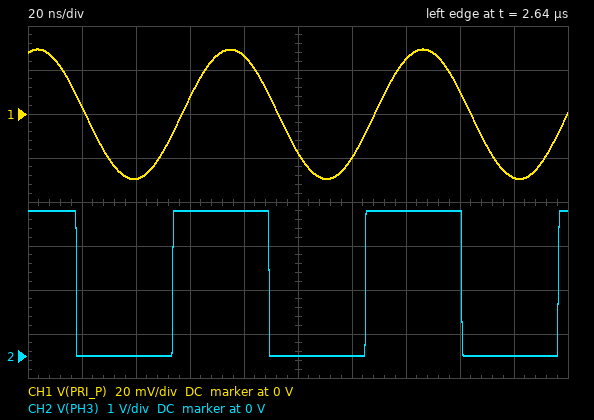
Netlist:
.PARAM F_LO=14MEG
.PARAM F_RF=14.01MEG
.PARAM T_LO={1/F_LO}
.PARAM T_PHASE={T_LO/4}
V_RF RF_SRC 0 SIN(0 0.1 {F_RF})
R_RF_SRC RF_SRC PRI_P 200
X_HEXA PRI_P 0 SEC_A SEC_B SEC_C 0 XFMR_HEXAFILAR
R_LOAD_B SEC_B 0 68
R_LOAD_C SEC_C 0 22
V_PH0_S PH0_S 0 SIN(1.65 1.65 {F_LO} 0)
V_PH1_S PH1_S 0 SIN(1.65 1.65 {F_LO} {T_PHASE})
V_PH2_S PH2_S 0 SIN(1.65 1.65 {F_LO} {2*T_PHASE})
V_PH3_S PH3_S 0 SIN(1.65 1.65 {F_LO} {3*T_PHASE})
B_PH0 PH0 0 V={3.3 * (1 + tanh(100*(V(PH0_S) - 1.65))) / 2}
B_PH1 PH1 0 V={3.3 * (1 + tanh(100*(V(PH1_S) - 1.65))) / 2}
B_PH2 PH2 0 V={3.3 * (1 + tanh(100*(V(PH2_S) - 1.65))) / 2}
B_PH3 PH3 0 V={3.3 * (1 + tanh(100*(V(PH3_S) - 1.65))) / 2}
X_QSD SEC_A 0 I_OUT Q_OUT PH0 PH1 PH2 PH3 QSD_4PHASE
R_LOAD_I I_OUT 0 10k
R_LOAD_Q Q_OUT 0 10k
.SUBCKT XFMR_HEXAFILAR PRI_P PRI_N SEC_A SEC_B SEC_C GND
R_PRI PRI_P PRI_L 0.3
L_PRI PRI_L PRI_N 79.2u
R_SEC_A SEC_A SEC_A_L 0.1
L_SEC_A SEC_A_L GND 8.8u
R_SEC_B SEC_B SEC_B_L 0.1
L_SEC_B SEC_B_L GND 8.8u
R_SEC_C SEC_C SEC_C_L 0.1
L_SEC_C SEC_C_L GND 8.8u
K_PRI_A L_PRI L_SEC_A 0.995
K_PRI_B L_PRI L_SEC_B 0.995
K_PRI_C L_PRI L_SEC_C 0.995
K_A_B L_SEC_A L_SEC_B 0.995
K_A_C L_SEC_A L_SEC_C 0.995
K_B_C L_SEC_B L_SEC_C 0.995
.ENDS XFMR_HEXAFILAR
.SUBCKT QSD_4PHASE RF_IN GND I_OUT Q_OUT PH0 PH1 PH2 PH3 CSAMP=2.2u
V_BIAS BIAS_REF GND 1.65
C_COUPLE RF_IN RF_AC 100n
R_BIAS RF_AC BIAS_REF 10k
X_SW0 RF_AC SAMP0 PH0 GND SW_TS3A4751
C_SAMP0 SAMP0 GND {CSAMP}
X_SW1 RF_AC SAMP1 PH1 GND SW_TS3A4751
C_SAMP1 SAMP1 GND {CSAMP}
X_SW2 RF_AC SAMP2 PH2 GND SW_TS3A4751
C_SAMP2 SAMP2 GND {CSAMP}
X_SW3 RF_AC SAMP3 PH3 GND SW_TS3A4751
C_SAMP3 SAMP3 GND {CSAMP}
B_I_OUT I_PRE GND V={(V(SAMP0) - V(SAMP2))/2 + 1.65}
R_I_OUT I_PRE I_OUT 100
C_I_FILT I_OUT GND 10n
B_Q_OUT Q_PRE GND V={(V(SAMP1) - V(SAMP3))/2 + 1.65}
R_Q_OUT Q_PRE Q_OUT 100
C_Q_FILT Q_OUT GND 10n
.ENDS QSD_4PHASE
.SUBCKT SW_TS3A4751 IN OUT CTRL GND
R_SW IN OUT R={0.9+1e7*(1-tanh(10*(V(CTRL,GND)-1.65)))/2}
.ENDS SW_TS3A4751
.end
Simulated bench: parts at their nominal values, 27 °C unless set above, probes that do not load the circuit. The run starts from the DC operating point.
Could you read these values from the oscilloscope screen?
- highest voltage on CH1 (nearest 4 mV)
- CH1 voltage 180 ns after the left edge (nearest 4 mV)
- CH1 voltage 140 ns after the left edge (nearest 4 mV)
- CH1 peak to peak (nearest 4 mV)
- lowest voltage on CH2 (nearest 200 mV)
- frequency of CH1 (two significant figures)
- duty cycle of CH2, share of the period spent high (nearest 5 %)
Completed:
28 mV
-28 mV
24 mV
60 mV
0 V
14 MHz
50 %
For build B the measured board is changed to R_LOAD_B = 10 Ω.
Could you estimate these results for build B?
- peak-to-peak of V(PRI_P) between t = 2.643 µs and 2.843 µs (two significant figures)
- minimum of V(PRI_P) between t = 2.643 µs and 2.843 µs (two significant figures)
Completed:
53 mV
-27 mV
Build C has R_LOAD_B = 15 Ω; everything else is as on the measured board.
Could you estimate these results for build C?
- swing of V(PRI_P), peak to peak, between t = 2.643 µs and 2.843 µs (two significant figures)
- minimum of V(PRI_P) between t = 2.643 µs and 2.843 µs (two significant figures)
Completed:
55 mV
-28 mV
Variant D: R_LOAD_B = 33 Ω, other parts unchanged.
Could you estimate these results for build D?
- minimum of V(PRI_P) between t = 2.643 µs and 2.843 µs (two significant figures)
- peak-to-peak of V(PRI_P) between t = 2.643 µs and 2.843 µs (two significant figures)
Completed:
-29 mV
58 mV
